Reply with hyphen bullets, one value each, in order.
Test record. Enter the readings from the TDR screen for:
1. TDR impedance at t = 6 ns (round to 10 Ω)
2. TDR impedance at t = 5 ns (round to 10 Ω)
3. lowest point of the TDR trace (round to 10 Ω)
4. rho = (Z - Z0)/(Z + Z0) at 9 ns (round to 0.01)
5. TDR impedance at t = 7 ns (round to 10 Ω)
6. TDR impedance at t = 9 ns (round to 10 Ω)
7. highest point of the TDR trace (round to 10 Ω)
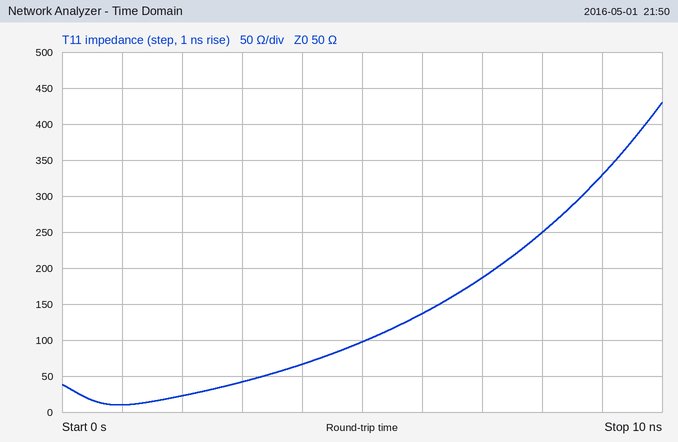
- 140 Ω
- 100 Ω
- 10 Ω
- +0.74
- 190 Ω
- 330 Ω
- 430 Ω
